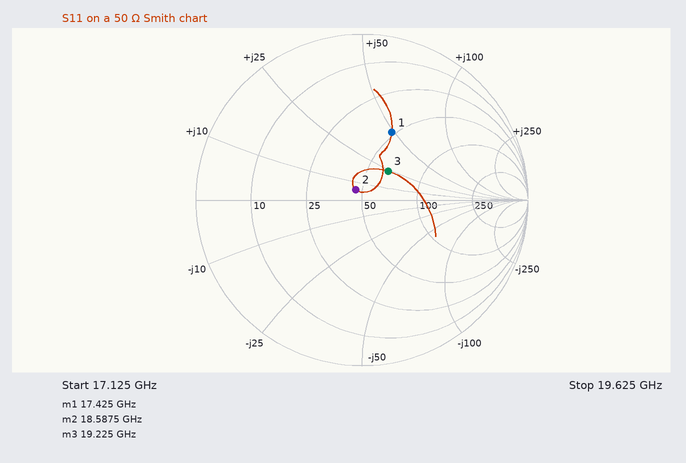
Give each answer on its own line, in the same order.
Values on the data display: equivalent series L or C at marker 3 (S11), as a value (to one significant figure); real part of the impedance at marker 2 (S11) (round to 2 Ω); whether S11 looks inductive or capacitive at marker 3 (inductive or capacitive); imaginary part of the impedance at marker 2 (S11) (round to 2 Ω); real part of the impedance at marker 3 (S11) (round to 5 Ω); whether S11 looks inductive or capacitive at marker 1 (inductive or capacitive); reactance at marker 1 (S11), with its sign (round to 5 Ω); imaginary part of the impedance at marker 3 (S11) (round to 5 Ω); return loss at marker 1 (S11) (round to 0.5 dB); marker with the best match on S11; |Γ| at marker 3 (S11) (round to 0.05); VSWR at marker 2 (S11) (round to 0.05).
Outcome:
200 pH
46 Ω
inductive
+6 Ω
65 Ω
inductive
+50 Ω
+25 Ω
7.0 dB
marker 2
0.25
1.15
